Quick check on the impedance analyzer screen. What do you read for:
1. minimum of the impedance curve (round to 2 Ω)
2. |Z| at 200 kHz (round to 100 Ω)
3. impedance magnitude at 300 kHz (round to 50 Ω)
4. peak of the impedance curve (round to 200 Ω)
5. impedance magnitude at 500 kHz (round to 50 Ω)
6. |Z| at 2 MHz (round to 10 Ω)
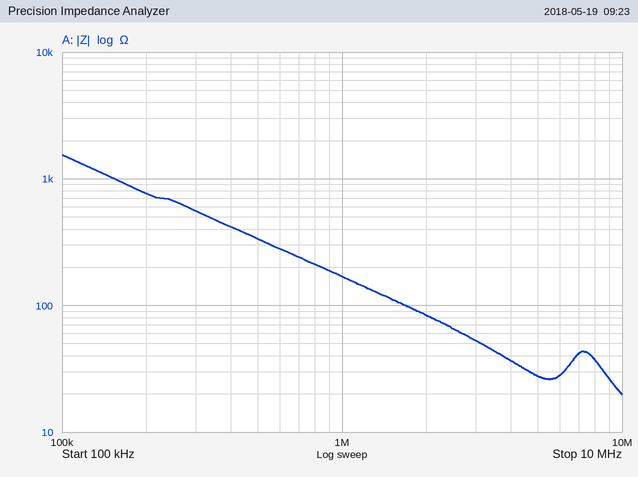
20 Ω
800 Ω
550 Ω
1.6 kΩ
350 Ω
80 Ω
